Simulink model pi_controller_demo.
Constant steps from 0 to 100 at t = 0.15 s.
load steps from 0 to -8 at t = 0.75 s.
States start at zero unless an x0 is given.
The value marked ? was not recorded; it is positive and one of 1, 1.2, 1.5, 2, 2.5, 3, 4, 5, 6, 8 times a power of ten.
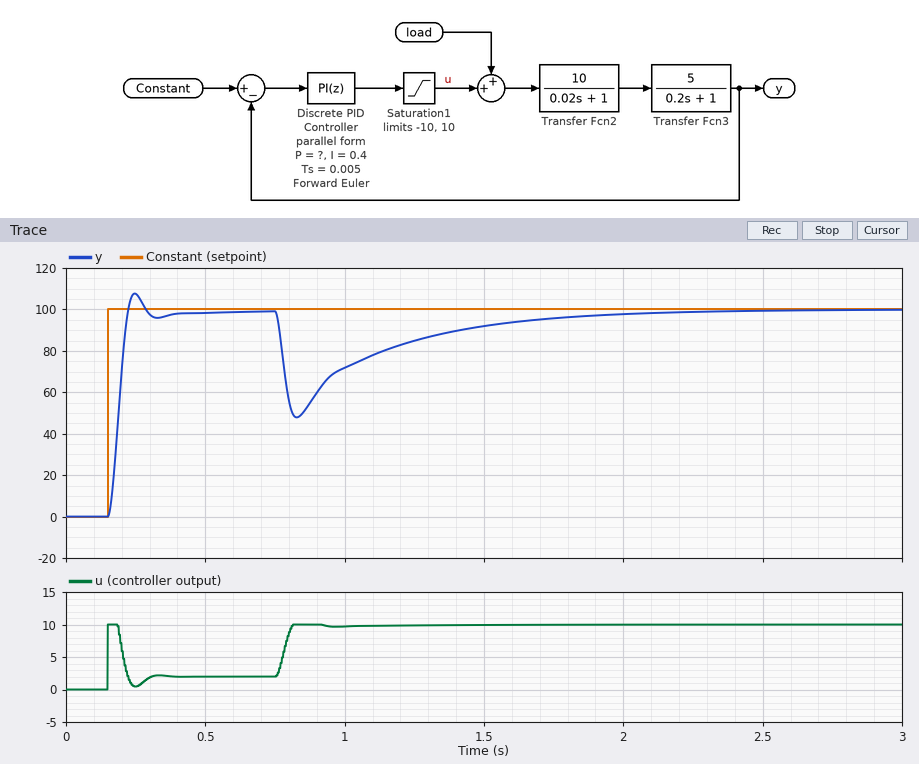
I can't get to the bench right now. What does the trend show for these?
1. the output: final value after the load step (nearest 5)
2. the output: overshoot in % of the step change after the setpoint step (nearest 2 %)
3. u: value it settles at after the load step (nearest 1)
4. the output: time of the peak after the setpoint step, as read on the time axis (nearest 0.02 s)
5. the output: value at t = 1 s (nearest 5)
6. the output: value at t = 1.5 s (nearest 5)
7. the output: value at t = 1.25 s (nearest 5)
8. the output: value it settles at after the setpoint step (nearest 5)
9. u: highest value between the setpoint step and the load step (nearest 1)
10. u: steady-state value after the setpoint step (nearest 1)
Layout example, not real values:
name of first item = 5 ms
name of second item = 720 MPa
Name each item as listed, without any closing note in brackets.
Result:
the output: final value after the load step = 100
the output: overshoot in % of the step change after the setpoint step = 8 %
u: value it settles at after the load step = 10
the output: time of the peak after the setpoint step, as read on the time axis = 0.24 s
the output: value at t = 1 s = 70
the output: value at t = 1.5 s = 90
the output: value at t = 1.25 s = 85
the output: value it settles at after the setpoint step = 100
u: highest value between the setpoint step and the load step = 10
u: steady-state value after the setpoint step = 2
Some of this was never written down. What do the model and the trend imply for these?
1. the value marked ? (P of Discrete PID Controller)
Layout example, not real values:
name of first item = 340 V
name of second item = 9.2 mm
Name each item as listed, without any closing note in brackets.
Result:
the value marked ? = 0.15
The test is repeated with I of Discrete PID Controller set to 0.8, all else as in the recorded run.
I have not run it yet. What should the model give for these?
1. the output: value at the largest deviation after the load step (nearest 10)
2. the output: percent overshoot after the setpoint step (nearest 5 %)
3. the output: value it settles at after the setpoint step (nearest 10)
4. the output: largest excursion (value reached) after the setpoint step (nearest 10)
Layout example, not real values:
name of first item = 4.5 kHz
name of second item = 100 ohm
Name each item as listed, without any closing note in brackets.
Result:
the output: value at the largest deviation after the load step = 50
the output: percent overshoot after the setpoint step = 15 %
the output: value it settles at after the setpoint step = 100
the output: largest excursion (value reached) after the setpoint step = 120
